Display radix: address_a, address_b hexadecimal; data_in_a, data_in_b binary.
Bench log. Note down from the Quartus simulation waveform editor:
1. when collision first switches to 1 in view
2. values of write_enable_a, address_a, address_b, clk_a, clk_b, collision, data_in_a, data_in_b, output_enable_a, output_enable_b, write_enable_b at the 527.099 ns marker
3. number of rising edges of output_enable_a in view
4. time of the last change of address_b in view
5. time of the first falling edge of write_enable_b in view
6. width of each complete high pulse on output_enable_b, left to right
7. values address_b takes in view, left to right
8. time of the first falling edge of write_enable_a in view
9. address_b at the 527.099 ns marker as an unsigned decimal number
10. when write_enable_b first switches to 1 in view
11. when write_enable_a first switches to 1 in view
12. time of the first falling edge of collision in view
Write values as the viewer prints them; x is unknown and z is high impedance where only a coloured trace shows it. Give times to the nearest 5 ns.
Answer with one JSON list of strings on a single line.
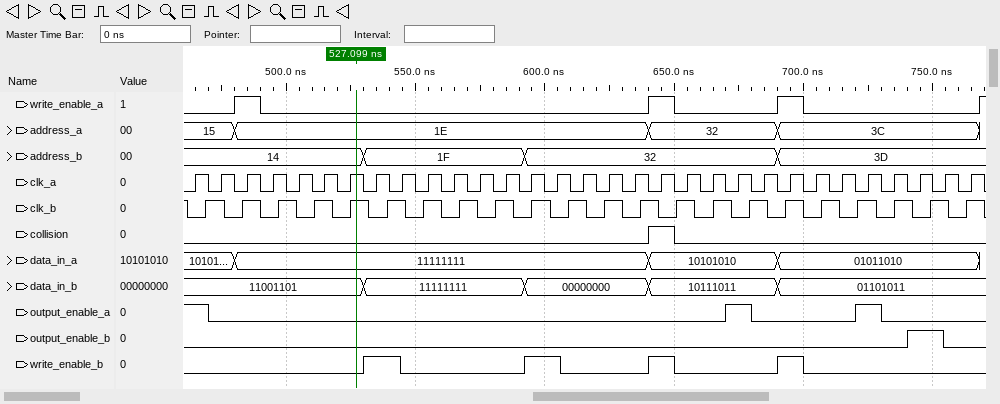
["640 ns", "write_enable_a=0, address_a=1E, address_b=14, clk_a=1, clk_b=1, collision=0, data_in_a=11111111, data_in_b=11001101, output_enable_a=0, output_enable_b=0, write_enable_b=0", "2", "690 ns", "545 ns", "15 ns", "14, 1F, 32, 3D", "490 ns", "20", "530 ns", "480 ns", "650 ns"]
